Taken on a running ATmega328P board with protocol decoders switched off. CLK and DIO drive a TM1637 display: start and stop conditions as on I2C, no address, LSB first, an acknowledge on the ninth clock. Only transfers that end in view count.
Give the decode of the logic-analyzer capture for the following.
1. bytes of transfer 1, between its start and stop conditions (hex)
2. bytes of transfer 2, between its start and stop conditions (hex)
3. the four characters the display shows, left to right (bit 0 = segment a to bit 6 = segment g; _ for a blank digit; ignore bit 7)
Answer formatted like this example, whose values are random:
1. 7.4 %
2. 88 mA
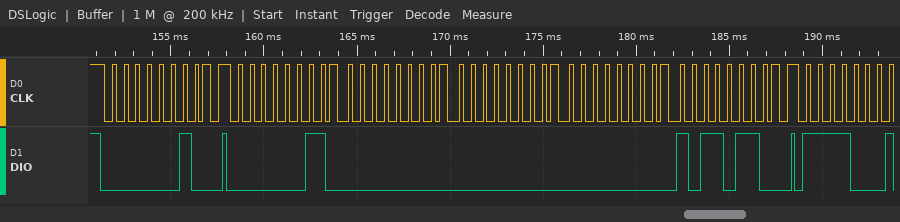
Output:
1. 40
2. C0 00 00 00 6D
3. ___5
